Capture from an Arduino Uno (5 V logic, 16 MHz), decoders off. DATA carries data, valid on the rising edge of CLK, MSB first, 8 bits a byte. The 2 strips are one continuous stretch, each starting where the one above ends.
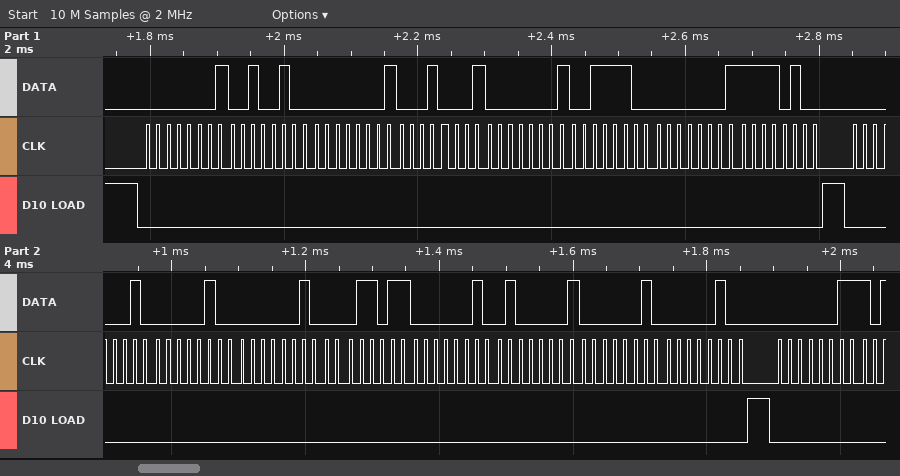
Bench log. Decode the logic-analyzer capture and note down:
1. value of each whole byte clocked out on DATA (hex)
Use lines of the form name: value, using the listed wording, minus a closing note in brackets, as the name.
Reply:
value of each whole byte clocked out on DATA: 01 24 01 11 01 3C 01 F4 02 04 02 1B 02 41 02 04 03
